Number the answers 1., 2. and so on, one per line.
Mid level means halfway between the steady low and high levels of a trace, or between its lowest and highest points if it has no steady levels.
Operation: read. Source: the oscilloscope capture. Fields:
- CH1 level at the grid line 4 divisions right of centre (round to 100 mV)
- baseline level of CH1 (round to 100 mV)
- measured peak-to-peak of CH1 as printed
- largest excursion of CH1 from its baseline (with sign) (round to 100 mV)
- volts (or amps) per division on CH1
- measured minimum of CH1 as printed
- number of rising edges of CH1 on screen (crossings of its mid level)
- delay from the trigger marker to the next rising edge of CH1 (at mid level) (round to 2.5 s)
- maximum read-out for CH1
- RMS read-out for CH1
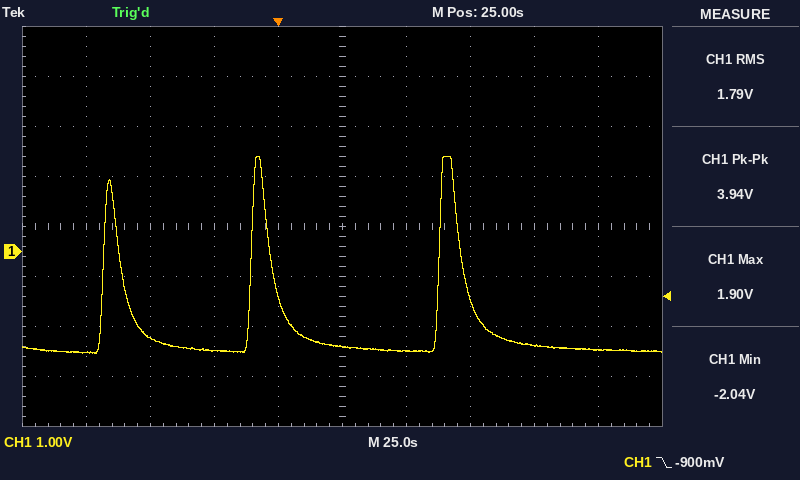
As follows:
1. -2.0 V
2. -2.0 V
3. 3.94 V
4. +3.9 V
5. 1 V
6. -2.04 V
7. 3
8. 62.5 s
9. 1.90 V
10. 1.79 V
